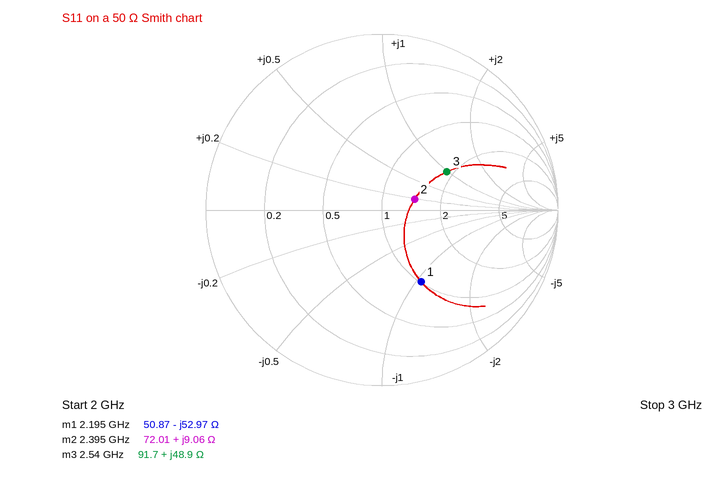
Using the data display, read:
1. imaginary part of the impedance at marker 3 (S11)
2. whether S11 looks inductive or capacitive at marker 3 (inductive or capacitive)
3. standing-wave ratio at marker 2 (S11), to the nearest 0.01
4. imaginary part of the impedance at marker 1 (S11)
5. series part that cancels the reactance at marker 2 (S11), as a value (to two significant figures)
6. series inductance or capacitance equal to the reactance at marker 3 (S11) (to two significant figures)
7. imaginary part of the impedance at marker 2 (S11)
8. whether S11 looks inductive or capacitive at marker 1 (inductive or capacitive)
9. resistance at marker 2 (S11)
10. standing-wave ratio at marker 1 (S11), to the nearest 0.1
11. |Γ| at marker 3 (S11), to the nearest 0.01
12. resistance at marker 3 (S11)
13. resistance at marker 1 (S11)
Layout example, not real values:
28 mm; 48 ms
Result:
+48.9 Ω; inductive; 1.48; -52.97 Ω; 7.3 pF; 3.1 nH; +9.06 Ω; capacitive; 72.01 Ω; 2.7; 0.43; 91.7 Ω; 50.87 Ω
